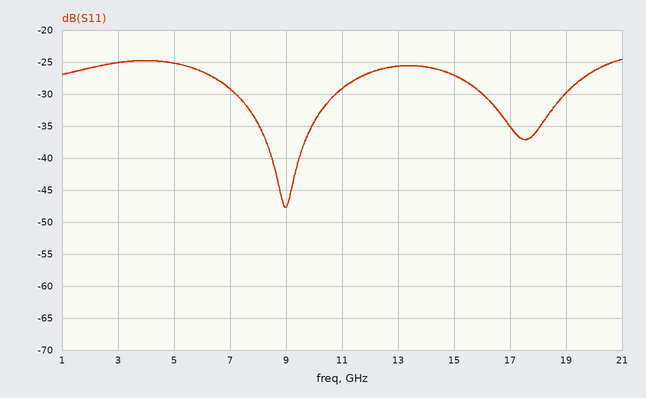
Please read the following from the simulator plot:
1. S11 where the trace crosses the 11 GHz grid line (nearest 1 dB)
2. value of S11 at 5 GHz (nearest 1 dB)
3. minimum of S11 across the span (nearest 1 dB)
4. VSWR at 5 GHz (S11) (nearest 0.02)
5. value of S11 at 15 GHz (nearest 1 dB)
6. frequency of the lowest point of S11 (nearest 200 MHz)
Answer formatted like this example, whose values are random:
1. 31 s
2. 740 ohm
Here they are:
1. -29 dB
2. -25 dB
3. -48 dB
4. 1.12
5. -27 dB
6. 9.0 GHz
